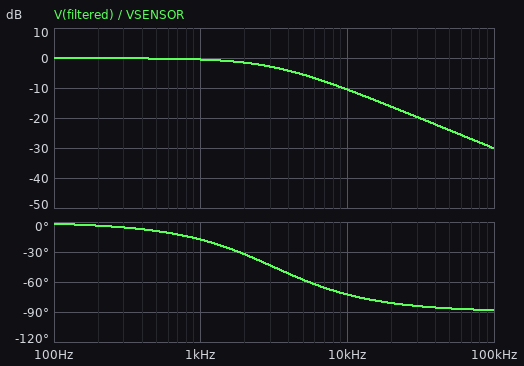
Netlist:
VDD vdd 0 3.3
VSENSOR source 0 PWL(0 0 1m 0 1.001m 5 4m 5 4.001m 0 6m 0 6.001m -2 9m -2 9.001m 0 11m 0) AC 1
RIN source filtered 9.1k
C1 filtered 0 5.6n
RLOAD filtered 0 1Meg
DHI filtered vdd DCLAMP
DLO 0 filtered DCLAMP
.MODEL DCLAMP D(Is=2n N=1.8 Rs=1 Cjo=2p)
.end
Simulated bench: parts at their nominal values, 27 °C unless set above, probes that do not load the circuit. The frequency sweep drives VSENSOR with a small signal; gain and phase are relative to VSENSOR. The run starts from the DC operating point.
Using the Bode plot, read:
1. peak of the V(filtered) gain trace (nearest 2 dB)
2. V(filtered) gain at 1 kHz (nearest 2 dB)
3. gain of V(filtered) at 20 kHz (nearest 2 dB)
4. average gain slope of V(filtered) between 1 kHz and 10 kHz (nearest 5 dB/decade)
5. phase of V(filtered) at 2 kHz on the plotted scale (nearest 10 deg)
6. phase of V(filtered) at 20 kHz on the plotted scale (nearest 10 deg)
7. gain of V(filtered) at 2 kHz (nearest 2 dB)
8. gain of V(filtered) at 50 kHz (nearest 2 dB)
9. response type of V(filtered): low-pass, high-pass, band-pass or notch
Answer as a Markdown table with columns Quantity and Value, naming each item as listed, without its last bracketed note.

| Quantity | Value |
|---|---|
| peak of the V(filtered) gain trace | 0 dB |
| V(filtered) gain at 1 kHz | 0 dB |
| gain of V(filtered) at 20 kHz | -16 dB |
| average gain slope of V(filtered) between 1 kHz and 10 kHz | -10 dB/decade |
| phase of V(filtered) at 2 kHz on the plotted scale | -30 deg |
| phase of V(filtered) at 20 kHz on the plotted scale | -80 deg |
| gain of V(filtered) at 2 kHz | -2 dB |
| gain of V(filtered) at 50 kHz | -24 dB |
| response type of V(filtered): low-pass, high-pass, band-pass or notch | low-pass |
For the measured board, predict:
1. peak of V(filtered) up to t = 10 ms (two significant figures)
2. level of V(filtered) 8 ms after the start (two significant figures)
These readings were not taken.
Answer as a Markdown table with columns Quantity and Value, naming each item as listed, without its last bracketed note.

| Quantity | Value |
|---|---|
| peak of V(filtered) up to t = 10 ms | 3.8 V |
| level of V(filtered) 8 ms after the start | -530 mV |
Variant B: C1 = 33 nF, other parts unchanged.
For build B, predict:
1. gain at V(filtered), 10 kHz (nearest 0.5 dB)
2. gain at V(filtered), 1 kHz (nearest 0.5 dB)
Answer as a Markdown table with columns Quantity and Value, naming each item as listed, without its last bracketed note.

| Quantity | Value |
|---|---|
| gain at V(filtered), 10 kHz | -25.5 dB |
| gain at V(filtered), 1 kHz | -6.5 dB |
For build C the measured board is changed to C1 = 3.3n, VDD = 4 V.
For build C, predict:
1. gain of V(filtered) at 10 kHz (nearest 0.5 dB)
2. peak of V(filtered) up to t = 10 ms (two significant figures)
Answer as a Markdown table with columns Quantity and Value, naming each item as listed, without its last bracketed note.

| Quantity | Value |
|---|---|
| gain of V(filtered) at 10 kHz | -6.5 dB |
| peak of V(filtered) up to t = 10 ms | 4.5 V |
